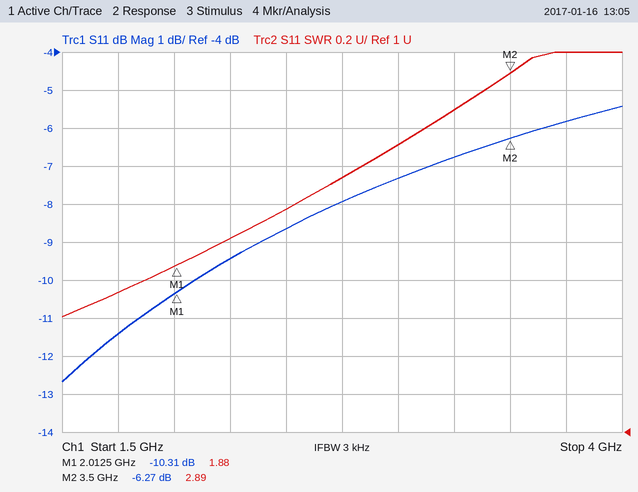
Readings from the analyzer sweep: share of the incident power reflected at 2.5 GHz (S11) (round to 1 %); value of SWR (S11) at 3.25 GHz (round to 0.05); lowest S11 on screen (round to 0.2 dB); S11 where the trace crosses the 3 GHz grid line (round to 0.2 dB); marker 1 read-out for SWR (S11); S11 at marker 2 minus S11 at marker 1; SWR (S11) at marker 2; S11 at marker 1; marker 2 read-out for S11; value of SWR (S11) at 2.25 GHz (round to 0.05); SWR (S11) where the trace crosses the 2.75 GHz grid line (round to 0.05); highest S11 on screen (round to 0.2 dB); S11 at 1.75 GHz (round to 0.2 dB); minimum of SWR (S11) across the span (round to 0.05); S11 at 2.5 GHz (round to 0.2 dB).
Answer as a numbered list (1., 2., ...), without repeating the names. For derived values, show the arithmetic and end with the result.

1. 10^(-8.6/10) ≈ 14 %
2. 2.70
3. -12.6 dB
4. -7.4 dB
5. 1.88
6. -6.27 − (-10.31) = 4.04 dB
7. 2.89
8. -10.31 dB
9. -6.27 dB
10. 2.00
11. 2.35
12. -5.4 dB
13. -11.4 dB
14. 1.60
15. -8.6 dB
